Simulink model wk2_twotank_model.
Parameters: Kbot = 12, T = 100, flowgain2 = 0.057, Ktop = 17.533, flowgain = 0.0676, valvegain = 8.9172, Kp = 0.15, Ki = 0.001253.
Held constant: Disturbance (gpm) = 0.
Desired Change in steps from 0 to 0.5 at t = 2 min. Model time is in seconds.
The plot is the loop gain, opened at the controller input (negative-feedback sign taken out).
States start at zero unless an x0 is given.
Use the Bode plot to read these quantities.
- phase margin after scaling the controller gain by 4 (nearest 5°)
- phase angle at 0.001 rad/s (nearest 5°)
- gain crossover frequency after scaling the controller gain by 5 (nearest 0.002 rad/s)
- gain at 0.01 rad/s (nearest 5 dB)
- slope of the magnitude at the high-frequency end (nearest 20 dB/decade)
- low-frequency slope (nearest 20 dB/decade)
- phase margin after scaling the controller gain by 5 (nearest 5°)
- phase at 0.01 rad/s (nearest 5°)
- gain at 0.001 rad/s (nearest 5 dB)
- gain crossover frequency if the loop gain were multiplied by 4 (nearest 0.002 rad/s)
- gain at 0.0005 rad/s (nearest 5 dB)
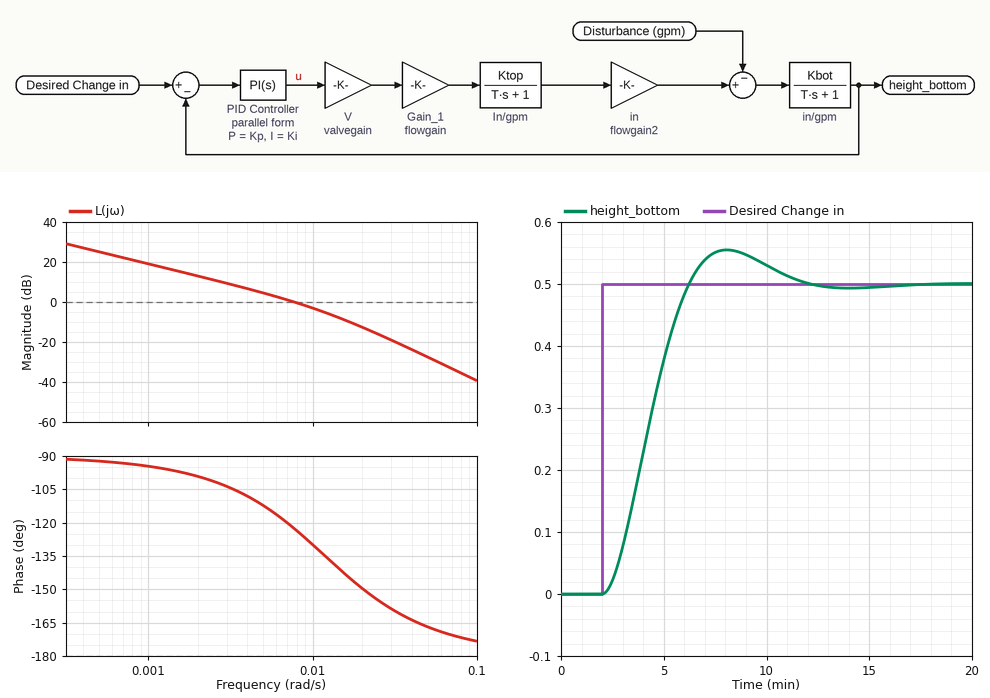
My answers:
30°
-95°
0.022 rad/s
-5 dB
-40 dB/decade
-20 dB/decade
30°
-130°
20 dB
0.020 rad/s
25 dB
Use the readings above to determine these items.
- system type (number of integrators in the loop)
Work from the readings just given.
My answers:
1
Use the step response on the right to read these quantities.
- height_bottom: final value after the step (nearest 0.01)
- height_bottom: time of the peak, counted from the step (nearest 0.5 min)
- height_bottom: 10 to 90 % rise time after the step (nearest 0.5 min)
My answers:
0.50
6.0 min
3.0 min
